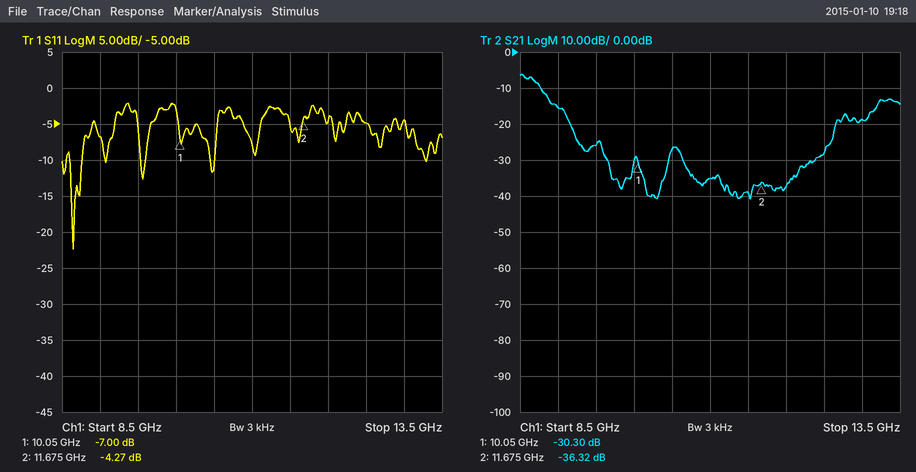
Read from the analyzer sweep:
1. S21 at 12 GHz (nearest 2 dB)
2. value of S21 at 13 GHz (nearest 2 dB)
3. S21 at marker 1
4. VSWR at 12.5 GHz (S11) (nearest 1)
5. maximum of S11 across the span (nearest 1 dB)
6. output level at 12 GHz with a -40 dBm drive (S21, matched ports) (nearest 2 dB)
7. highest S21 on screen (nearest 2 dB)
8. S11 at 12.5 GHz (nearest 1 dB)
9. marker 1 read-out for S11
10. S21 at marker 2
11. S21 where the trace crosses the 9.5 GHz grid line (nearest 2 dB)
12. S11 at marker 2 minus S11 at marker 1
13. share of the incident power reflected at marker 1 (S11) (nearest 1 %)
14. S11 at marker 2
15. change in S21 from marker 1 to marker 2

-38 dB
-18 dB
-30.30 dB
4
-2 dB
-78 dBm
-6 dB
-5 dB
-7.00 dB
-36.32 dB
-26 dB
2.73 dB
20 %
-4.27 dB
-6.02 dB
